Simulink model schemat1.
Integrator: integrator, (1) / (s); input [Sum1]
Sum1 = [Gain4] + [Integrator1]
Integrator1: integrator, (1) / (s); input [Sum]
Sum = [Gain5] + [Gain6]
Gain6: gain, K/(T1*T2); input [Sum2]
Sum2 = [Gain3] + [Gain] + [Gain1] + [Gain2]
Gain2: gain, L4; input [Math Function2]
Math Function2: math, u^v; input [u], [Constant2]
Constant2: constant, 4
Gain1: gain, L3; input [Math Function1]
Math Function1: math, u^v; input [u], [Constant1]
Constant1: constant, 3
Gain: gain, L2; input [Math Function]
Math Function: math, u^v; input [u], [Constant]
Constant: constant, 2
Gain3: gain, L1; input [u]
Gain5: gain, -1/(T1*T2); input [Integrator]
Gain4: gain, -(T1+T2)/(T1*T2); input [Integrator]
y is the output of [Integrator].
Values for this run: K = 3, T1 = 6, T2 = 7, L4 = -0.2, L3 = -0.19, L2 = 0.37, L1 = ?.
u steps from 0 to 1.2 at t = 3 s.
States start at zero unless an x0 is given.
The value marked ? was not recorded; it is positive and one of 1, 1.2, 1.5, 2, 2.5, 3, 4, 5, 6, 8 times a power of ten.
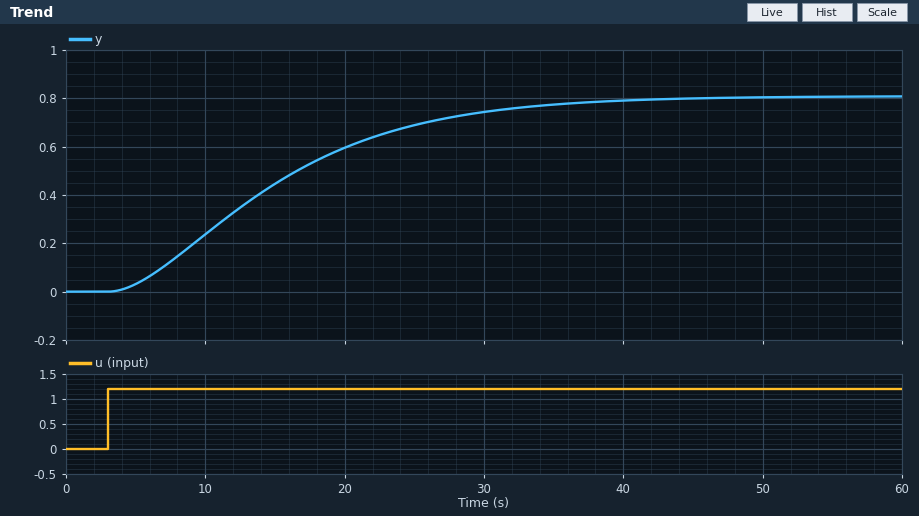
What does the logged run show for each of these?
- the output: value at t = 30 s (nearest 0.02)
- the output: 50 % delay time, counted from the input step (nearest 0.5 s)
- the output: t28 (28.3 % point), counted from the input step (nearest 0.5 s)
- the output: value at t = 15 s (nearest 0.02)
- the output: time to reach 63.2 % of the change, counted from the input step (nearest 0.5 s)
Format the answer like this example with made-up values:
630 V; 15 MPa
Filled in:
0.74; 11.0 s; 7.0 s; 0.44; 14.0 s
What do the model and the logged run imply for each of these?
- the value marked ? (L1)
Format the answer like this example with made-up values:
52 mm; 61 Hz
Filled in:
0.4
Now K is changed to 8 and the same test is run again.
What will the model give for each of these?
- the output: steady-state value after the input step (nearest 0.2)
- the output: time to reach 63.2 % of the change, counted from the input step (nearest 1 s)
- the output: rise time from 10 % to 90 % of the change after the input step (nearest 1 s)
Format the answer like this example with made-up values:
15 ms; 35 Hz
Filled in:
2.2; 14 s; 22 s
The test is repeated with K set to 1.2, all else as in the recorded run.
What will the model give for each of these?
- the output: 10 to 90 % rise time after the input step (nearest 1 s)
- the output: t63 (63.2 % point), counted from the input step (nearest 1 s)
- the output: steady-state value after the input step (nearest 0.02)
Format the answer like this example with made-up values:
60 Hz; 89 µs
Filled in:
22 s; 14 s; 0.32
